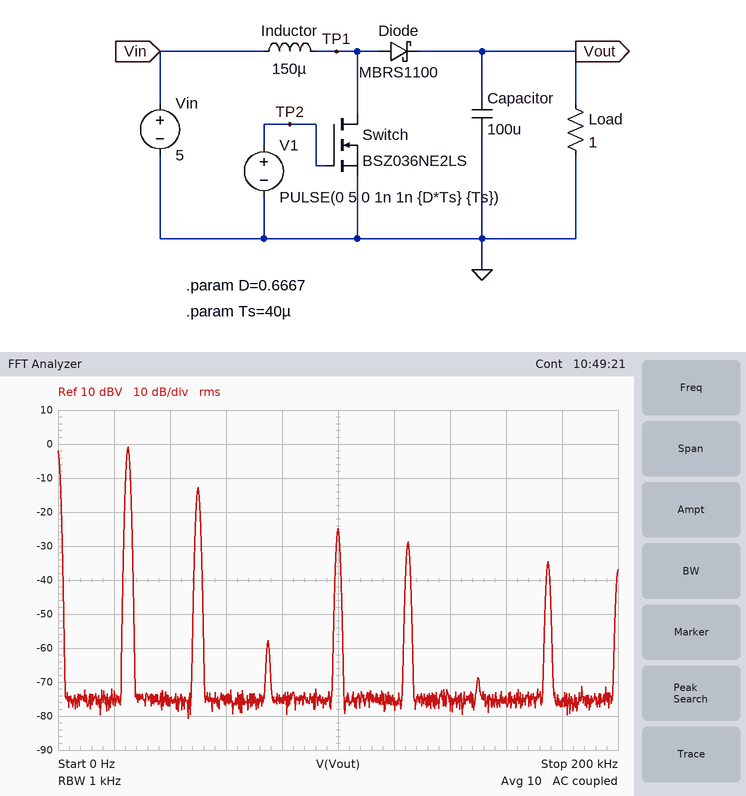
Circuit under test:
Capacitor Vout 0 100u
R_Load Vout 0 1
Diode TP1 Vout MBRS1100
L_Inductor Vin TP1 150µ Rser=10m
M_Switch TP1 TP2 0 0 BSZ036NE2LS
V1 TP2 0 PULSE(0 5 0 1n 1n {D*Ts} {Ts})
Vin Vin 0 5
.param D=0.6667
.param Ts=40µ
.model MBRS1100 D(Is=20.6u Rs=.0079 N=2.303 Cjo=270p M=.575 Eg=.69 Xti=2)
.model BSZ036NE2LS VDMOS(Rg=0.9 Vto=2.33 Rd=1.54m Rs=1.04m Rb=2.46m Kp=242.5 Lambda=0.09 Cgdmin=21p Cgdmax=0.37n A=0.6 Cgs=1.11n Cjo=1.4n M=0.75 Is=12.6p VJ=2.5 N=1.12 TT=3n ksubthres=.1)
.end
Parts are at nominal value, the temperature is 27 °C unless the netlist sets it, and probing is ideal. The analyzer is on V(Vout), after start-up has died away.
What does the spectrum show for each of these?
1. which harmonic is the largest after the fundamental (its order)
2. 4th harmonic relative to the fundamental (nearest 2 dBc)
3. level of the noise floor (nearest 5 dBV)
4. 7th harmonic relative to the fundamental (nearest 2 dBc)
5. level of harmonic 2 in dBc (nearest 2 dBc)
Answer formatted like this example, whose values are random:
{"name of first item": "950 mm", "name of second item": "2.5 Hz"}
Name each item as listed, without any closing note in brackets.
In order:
{"which harmonic is the largest after the fundamental": "2", "4th harmonic relative to the fundamental": "-24 dBc", "level of the noise floor": "-75 dBV", "7th harmonic relative to the fundamental": "-34 dBc", "level of harmonic 2 in dBc": "-12 dBc"}
